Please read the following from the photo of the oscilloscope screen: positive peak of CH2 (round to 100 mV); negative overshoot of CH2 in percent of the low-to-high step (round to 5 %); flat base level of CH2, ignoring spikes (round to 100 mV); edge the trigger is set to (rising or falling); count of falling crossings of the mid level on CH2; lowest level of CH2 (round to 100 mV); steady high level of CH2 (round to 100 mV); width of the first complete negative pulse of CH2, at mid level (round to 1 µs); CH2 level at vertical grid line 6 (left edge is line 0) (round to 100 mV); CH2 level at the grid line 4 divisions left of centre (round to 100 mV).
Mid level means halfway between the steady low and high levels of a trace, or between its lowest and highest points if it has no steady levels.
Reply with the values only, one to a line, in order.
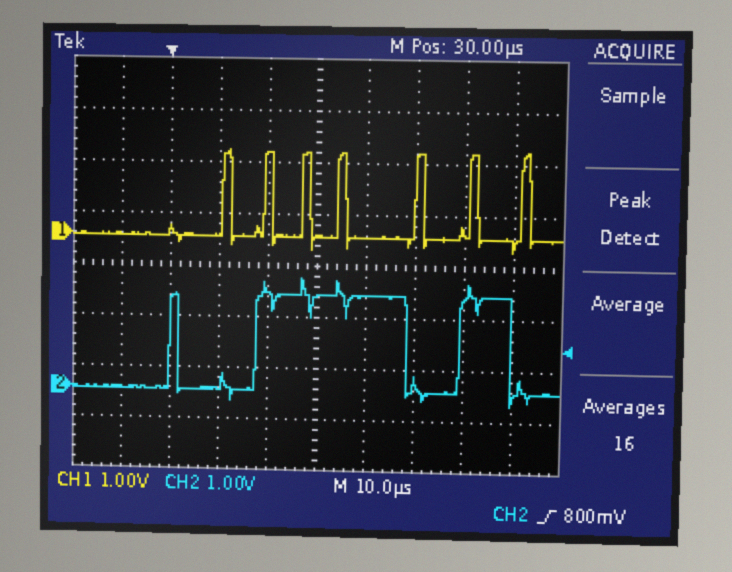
2.2 V
15 %
0.0 V
rising
3
-300 mV
1.8 V
16 µs
1.8 V
0.0 V
